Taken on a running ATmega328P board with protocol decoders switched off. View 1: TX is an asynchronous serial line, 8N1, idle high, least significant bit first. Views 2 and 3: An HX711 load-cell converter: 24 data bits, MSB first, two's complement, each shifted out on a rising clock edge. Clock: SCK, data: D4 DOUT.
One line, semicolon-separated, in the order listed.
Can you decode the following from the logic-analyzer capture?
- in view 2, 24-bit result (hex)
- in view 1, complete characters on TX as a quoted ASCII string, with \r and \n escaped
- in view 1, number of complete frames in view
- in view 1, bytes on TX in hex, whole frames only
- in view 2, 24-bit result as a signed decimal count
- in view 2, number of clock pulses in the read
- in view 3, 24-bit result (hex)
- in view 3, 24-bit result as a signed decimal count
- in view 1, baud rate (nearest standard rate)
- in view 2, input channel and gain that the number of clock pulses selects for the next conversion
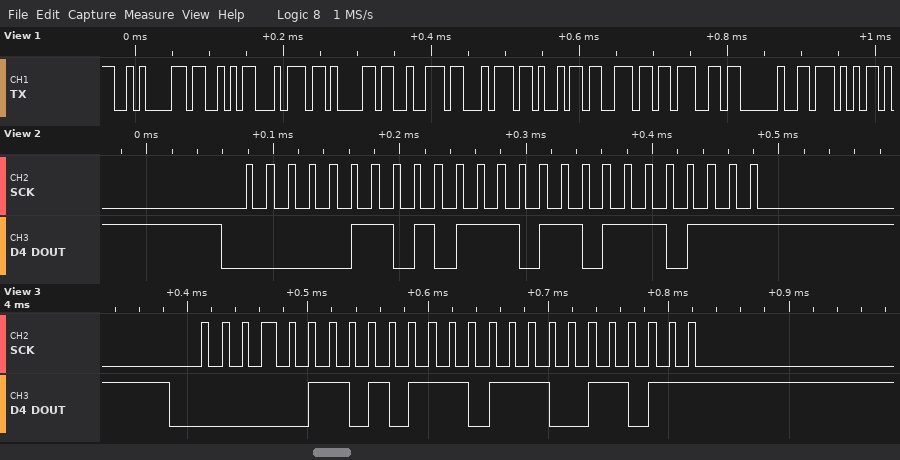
0x06BB77; "\nStarting W"; 11; 0A 53 74 61 72 74 69 6E 67 20 57; 441207; 25; 0x06BB9B; 441243; 115200 baud; channel A, gain 128
